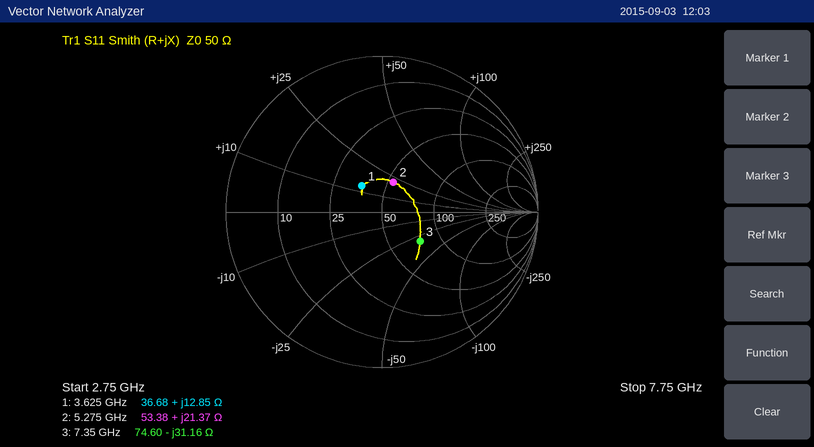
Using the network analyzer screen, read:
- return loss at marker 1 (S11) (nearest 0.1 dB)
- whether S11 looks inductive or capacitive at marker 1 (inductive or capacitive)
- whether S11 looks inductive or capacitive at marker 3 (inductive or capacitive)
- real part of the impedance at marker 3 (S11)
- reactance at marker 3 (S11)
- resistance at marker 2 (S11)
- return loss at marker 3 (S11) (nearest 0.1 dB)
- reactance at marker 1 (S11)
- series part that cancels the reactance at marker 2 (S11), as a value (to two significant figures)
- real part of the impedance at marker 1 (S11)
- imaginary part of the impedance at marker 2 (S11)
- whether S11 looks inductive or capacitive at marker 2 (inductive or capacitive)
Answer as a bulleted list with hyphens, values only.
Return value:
- 13.5 dB
- inductive
- capacitive
- 74.60 Ω
- -31.16 Ω
- 53.38 Ω
- 10.2 dB
- +12.85 Ω
- 1.4 pF
- 36.68 Ω
- +21.37 Ω
- inductive
